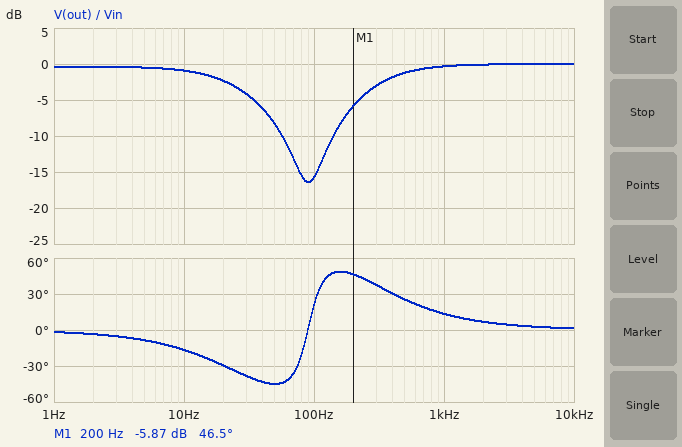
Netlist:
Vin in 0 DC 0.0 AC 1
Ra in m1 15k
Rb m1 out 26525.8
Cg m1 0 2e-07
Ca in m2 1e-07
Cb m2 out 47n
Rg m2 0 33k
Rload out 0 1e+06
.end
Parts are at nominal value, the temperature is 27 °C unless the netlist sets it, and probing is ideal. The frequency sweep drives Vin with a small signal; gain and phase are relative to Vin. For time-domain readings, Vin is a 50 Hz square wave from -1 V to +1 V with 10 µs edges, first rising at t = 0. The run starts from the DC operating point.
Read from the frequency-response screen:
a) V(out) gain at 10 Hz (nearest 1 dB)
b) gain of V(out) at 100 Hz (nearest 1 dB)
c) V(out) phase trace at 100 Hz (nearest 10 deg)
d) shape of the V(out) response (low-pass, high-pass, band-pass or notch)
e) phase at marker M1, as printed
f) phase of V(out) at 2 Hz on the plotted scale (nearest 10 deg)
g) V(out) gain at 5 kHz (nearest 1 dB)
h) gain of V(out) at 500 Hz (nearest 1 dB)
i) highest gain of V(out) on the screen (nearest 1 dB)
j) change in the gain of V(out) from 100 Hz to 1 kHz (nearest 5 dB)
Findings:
-1 dB
-16 dB
20 deg
notch
46.5 deg
0 deg
0 dB
-1 dB
0 dB
15 dB
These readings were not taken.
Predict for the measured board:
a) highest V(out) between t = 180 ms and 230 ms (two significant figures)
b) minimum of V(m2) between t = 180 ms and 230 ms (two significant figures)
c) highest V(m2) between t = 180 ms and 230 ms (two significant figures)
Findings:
1.3 V
-1.7 V
1.7 V
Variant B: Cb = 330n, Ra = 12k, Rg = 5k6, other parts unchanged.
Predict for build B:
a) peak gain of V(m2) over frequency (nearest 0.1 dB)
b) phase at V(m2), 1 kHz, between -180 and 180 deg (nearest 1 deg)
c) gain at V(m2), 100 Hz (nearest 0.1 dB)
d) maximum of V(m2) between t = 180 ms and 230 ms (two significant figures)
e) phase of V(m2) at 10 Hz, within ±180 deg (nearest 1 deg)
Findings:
0 dB
19 deg
-12.2 dB
1.9 V
52 deg
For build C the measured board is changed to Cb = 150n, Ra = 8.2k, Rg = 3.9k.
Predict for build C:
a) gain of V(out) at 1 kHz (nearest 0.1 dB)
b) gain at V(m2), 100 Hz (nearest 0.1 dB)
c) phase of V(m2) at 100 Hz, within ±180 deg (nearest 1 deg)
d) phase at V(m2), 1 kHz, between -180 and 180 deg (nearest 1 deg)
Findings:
-1.0 dB
-13.9 dB
56 deg
25 deg
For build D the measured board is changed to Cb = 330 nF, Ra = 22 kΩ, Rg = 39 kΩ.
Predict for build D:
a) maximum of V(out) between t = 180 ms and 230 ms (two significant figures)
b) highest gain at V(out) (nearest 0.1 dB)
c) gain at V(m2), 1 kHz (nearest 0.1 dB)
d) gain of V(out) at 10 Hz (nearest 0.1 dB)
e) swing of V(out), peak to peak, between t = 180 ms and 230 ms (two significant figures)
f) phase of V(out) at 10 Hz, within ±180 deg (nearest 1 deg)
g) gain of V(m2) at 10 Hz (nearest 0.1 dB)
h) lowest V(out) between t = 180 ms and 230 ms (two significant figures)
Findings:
1.6 V
0 dB
-0.1 dB
-5.5 dB
3.2 V
-28 deg
-6.9 dB
-1.6 V
